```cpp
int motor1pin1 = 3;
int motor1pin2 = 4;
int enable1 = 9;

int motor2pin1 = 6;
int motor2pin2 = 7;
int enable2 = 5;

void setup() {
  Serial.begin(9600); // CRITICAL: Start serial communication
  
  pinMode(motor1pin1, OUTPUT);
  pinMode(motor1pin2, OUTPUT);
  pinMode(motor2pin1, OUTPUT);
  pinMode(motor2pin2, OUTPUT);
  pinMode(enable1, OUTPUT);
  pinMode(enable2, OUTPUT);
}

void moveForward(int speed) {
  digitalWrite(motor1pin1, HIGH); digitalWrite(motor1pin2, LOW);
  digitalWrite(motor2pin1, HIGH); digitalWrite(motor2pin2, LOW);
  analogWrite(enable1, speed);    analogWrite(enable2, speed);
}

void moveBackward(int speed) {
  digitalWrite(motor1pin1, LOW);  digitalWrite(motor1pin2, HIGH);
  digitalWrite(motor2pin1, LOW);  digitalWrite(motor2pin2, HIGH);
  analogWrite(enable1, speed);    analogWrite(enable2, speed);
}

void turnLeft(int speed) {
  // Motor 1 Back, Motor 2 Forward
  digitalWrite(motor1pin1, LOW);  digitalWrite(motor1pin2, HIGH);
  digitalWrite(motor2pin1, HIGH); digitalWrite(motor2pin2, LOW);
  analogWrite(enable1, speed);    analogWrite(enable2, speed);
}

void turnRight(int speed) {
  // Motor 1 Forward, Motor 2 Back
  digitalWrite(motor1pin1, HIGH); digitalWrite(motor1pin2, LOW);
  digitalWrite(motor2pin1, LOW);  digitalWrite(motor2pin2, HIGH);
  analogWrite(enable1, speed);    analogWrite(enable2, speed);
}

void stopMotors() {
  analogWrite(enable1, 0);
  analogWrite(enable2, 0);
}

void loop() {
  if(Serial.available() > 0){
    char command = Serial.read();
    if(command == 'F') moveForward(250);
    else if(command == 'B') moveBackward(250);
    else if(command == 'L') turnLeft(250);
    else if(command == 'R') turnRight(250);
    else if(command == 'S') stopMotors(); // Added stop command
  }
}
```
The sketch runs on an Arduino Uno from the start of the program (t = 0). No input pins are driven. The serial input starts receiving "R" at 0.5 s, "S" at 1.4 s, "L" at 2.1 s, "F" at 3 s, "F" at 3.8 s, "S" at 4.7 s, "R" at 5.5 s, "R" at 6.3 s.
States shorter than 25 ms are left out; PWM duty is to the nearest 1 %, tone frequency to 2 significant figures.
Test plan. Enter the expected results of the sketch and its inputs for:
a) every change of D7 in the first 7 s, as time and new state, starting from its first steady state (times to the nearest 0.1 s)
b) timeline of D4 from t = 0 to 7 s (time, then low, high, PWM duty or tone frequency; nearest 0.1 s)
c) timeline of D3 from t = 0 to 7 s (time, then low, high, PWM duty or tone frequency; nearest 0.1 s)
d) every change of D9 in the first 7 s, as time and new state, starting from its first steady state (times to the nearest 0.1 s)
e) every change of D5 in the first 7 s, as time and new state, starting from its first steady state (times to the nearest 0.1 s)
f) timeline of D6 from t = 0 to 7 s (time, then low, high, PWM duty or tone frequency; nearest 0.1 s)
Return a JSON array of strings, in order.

["0 s low; 0.5 s high; 2.1 s low; 5.5 s high", "0 s low; 2.1 s high; 3 s low", "0 s low; 0.5 s high; 2.1 s low; 3 s high", "0 s low; 0.5 s PWM 98 %; 1.4 s low; 2.1 s PWM 98 %; 4.7 s low; 5.5 s PWM 98 %", "0 s low; 0.5 s PWM 98 %; 1.4 s low; 2.1 s PWM 98 %; 4.7 s low; 5.5 s PWM 98 %", "0 s low; 2.1 s high; 5.5 s low"]
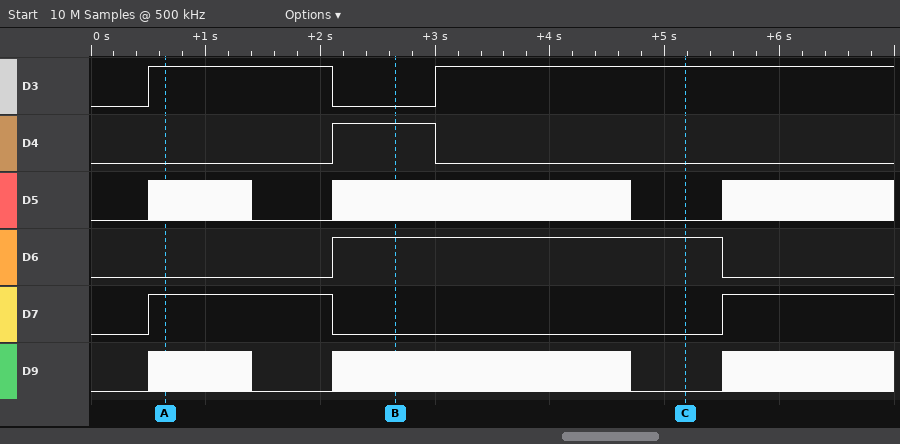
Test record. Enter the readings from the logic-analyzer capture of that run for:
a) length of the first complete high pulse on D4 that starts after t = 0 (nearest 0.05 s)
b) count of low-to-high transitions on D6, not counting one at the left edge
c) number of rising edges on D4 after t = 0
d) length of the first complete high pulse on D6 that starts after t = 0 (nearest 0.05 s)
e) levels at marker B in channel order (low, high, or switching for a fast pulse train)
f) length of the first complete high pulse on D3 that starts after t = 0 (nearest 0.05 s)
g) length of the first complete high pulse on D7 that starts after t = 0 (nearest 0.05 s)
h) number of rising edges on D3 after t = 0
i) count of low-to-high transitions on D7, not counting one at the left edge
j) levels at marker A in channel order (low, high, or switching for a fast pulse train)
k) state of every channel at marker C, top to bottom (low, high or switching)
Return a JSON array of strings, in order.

["0.90 s", "1", "1", "3.40 s", "D3 low, D4 high, D5 switching, D6 high, D7 low, D9 switching", "1.60 s", "1.60 s", "2", "2", "D3 high, D4 low, D5 switching, D6 low, D7 high, D9 switching", "D3 high, D4 low, D5 low, D6 high, D7 low, D9 low"]
